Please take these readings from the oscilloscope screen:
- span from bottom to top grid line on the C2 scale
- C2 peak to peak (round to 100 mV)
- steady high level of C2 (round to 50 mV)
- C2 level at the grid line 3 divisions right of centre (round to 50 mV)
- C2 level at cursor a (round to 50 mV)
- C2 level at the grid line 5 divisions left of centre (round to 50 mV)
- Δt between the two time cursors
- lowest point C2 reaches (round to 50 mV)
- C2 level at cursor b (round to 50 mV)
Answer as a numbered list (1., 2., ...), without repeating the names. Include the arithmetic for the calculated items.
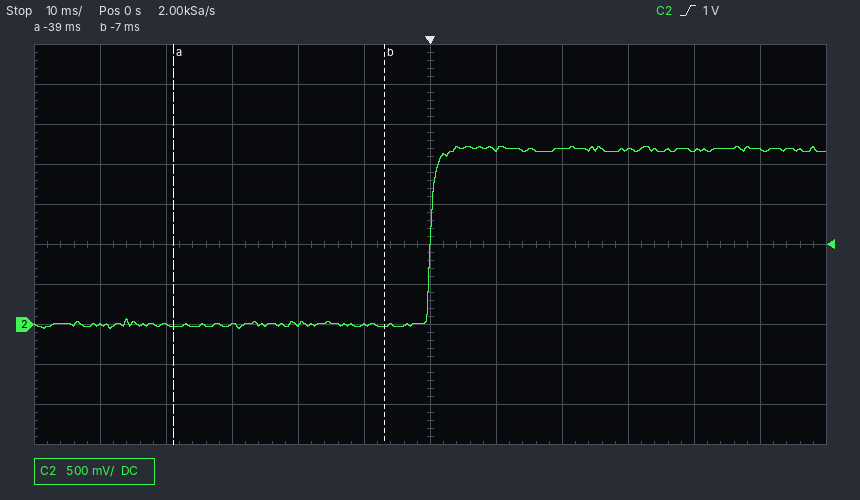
1. 5 V
2. 2.30 V
3. 2.20 V
4. 2.20 V
5. 0 mV
6. 0 mV
7. -7 ms − (-39 ms) = 32 ms
8. -50 mV
9. 0 mV
